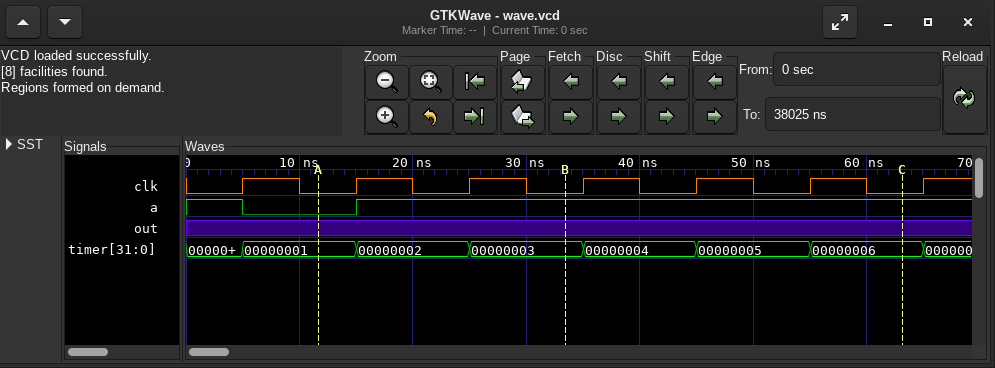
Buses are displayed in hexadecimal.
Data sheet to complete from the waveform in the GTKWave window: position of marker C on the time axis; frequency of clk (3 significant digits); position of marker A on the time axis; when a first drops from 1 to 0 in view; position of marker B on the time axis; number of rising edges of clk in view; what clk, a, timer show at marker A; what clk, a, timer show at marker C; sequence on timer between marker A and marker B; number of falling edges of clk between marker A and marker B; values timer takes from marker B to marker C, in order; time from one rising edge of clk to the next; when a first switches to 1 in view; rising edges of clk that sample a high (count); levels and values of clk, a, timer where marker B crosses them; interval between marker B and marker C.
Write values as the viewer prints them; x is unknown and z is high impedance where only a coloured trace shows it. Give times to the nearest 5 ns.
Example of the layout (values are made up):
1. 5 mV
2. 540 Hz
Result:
1. 65 ns
2. 100 MHz
3. 10 ns
4. 5 ns
5. 35 ns
6. 7
7. clk=0, a=0, timer=00000001
8. clk=0, a=1, timer=00000006
9. 00000001, 00000002, 00000003
10. 2
11. 00000003, 00000004, 00000005, 00000006
12. 10 ns
13. 15 ns
14. 6
15. clk=0, a=1, timer=00000003
16. 30 ns
